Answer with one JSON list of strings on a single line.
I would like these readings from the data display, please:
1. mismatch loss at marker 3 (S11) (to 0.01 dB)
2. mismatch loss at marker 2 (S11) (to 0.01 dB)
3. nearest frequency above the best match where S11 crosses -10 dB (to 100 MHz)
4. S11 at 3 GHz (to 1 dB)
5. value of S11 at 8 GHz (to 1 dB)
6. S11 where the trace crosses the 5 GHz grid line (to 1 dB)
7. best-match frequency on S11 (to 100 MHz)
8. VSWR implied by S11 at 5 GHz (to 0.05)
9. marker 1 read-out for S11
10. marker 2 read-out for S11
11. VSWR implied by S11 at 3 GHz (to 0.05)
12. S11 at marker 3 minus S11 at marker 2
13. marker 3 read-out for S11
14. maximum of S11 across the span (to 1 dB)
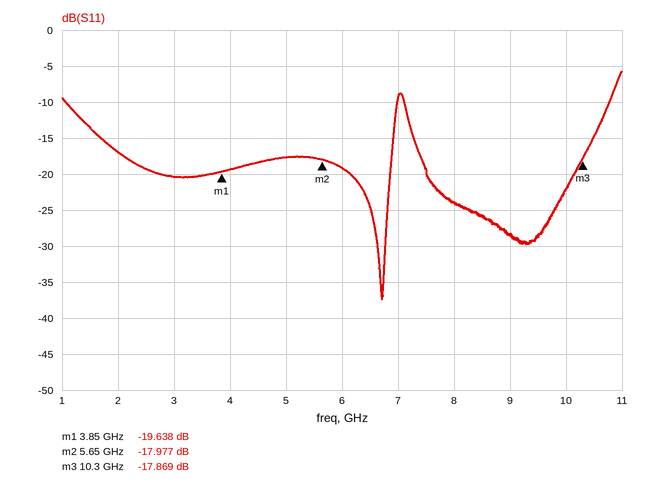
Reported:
["0.07 dB", "0.07 dB", "7.0 GHz", "-20 dB", "-24 dB", "-18 dB", "6.7 GHz", "1.30", "-19.638 dB", "-17.977 dB", "1.20", "0.108 dB", "-17.869 dB", "-6 dB"]
